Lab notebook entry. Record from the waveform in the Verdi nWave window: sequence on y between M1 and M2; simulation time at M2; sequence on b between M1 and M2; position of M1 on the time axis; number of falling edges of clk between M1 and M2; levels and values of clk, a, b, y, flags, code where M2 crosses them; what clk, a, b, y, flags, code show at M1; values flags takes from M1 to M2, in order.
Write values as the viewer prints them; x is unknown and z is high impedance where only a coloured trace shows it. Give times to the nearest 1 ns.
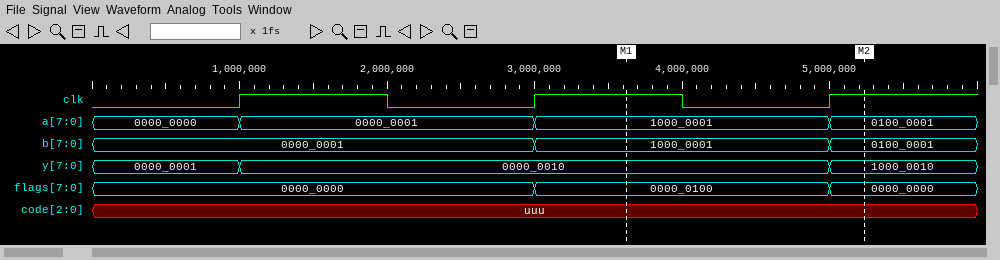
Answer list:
0000_0010, 1000_0010
5 ns
1000_0001, 0100_0001
4 ns
1
clk=1, a=0100_0001, b=0100_0001, y=1000_0010, flags=0000_0000, code=uuu
clk=1, a=1000_0001, b=1000_0001, y=0000_0010, flags=0000_0100, code=uuu
0000_0100, 0000_0000
